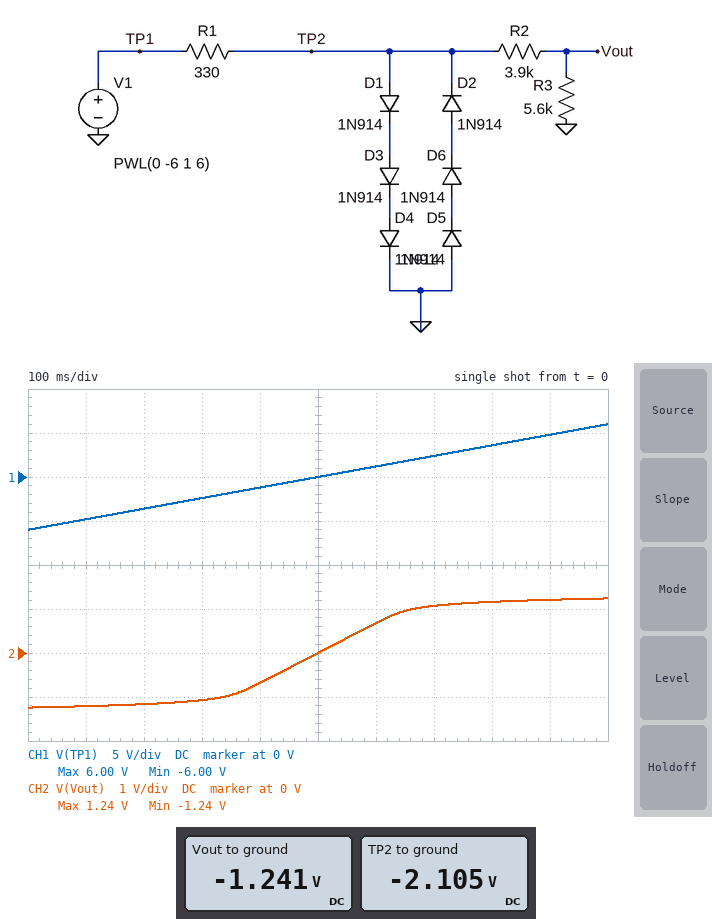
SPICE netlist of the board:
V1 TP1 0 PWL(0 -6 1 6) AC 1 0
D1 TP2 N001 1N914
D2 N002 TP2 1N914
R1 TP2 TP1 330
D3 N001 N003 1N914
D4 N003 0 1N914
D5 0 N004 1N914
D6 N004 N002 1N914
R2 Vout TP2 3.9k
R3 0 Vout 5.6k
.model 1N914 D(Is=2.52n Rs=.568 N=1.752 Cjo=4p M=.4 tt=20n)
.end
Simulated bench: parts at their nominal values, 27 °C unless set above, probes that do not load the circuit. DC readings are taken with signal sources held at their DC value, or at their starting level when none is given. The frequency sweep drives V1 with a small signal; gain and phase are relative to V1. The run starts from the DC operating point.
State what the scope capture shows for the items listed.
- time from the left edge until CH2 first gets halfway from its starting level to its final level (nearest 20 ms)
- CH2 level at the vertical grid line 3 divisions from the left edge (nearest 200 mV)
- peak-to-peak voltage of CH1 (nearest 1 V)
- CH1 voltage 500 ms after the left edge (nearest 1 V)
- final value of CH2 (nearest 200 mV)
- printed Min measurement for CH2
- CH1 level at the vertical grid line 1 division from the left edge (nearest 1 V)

500 ms
-1.0 V
12 V
0 V
1.2 V
-1.24 V
-5 V
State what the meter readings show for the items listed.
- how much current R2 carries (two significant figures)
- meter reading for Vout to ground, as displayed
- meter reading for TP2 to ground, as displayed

220 µA
-1.241 V
-2.105 V
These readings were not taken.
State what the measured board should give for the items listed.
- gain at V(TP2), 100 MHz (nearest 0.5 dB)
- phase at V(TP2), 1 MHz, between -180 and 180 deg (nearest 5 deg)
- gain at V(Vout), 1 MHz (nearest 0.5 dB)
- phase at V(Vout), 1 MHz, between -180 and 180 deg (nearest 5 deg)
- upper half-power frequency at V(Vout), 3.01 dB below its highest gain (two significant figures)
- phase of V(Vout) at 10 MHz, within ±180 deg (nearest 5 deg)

-44.5 dB
-5 deg
-33.0 dB
-5 deg
8.4 MHz
-40 deg
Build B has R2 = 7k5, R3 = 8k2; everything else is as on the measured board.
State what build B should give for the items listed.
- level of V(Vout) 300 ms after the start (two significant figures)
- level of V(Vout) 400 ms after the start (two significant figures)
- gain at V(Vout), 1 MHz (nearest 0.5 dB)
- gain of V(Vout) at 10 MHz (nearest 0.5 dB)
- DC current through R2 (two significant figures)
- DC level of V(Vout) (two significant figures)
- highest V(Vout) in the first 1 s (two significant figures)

-950 mV
-610 mV
-34.0 dB
-37.5 dB
130 µA
-1.1 V
1.1 V
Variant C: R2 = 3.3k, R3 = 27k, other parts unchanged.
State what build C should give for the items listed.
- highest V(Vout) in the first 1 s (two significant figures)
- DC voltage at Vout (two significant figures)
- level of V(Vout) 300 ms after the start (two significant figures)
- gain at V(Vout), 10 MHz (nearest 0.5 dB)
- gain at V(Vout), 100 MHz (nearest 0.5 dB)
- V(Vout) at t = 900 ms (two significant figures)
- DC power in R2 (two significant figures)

1.9 V
-1.9 V
-1.6 V
-33.0 dB
-45.5 dB
1.8 V
16 µW
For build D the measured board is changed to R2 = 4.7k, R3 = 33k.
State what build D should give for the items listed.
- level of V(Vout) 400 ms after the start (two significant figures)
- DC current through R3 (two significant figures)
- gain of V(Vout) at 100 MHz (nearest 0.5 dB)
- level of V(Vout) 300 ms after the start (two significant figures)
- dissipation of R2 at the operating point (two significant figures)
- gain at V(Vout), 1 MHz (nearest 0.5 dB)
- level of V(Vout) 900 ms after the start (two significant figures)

-1.0 V
56 µA
-45.5 dB
-1.6 V
15 µW
-29.5 dB
1.8 V
